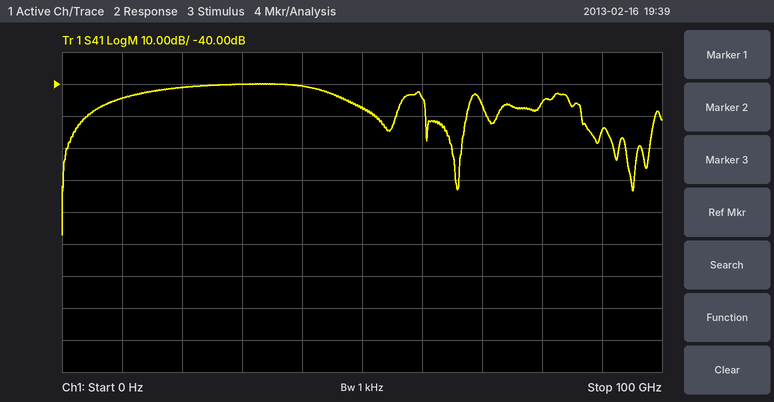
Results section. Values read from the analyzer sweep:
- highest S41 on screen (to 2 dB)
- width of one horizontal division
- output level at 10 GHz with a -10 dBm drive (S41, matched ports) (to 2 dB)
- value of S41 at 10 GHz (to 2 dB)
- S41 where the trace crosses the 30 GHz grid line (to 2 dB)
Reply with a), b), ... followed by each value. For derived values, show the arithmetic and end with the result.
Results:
a) -40 dB
b) 10 GHz
c) -10 dBm + (-44 dB) = -54 dBm
d) -44 dB
e) -40 dB
